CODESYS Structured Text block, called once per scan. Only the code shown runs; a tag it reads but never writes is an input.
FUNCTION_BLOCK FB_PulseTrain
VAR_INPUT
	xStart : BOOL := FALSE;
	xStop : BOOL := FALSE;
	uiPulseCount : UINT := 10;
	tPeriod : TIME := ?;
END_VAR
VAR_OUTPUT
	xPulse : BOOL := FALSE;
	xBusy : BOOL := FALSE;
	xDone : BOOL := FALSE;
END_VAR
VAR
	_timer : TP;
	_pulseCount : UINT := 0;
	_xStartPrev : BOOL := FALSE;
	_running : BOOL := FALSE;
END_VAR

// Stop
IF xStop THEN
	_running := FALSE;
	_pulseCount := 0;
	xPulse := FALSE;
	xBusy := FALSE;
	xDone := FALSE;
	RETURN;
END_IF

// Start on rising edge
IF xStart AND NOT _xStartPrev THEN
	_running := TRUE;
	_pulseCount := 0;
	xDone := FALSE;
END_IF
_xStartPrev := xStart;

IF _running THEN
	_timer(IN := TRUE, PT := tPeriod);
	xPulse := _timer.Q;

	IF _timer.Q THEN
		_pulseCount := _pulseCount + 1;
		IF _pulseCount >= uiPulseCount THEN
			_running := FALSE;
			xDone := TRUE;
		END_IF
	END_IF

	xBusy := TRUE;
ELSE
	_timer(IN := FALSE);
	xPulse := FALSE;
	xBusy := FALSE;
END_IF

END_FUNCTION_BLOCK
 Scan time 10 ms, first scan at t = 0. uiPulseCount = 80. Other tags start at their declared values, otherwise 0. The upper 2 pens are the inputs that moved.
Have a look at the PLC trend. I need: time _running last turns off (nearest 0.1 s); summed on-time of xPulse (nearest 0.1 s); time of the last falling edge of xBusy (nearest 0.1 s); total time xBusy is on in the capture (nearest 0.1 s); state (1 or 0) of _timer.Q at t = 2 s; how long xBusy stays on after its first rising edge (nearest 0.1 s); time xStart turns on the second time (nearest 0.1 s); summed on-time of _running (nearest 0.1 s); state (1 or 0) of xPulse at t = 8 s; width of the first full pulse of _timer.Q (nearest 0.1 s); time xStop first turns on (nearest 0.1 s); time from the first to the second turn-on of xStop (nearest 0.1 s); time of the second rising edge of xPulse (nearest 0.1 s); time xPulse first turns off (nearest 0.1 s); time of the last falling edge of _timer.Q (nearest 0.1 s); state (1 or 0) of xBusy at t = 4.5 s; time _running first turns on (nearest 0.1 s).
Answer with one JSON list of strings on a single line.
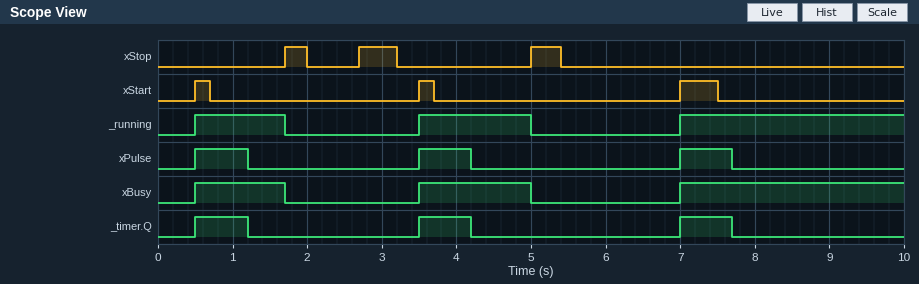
["5.0 s", "2.1 s", "5.0 s", "5.7 s", "0", "1.2 s", "3.5 s", "5.7 s", "0", "0.7 s", "1.7 s", "1.0 s", "3.5 s", "1.2 s", "7.7 s", "1", "0.5 s"]
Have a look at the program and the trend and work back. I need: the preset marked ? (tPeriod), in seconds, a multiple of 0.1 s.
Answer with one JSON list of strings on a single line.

["0.7 s"]
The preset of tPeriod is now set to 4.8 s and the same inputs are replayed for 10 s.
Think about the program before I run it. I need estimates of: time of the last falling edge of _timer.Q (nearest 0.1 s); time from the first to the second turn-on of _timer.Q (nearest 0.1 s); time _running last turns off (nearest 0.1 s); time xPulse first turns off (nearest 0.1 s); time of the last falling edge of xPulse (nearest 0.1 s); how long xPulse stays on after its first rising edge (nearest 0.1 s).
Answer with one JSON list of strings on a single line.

["5.4 s", "6.5 s", "7.8 s", "1.3 s", "7.8 s", "0.8 s"]
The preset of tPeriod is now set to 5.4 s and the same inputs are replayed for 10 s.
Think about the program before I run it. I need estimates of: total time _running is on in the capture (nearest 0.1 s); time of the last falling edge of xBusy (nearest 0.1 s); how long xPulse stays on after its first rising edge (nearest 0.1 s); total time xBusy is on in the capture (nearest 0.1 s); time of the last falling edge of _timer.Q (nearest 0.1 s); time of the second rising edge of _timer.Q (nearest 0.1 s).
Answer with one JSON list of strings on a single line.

["2.4 s", "7.8 s", "0.8 s", "2.4 s", "5.9 s", "7.0 s"]
